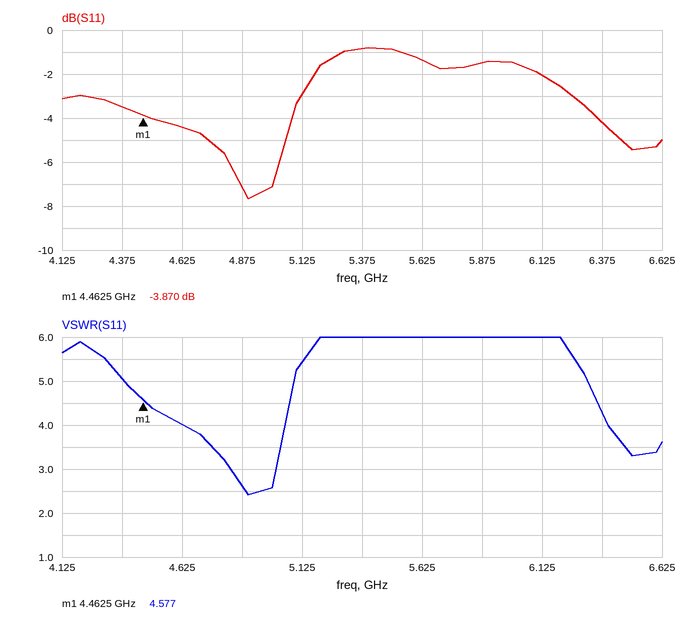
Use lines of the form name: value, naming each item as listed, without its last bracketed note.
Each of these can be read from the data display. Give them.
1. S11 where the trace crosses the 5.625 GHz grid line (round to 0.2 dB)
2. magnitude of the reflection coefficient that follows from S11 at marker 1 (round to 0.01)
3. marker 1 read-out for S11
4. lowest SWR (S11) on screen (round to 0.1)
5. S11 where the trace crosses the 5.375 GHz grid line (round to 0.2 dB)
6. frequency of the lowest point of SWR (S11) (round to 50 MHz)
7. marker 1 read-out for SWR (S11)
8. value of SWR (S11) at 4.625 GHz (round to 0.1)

S11 where the trace crosses the 5.625 GHz grid line: -1.4 dB
magnitude of the reflection coefficient that follows from S11 at marker 1: 0.64
marker 1 read-out for S11: -3.870 dB
lowest SWR (S11) on screen: 2.4
S11 where the trace crosses the 5.375 GHz grid line: -0.8 dB
frequency of the lowest point of SWR (S11): 4.90 GHz
marker 1 read-out for SWR: 4.577
value of SWR (S11) at 4.625 GHz: 4.0
